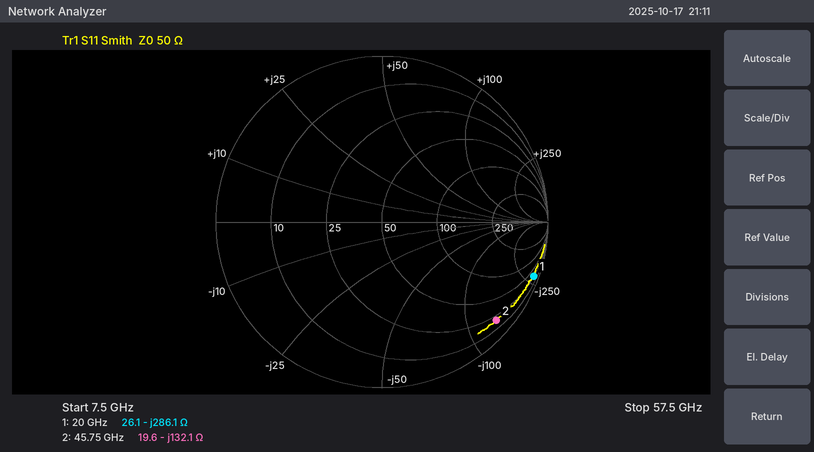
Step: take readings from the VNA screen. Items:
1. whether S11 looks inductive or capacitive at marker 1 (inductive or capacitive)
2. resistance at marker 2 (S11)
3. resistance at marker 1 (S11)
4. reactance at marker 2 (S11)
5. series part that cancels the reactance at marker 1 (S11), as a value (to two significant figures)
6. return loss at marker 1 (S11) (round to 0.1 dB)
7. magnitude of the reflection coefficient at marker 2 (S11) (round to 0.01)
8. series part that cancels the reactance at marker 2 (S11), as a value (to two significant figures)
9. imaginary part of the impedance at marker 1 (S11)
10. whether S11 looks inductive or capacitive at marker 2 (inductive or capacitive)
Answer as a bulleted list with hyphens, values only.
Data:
- capacitive
- 19.6 Ω
- 26.1 Ω
- -132.1 Ω
- 2.3 nH
- 0.3 dB
- 0.91
- 460 pH
- -286.1 Ω
- capacitive
